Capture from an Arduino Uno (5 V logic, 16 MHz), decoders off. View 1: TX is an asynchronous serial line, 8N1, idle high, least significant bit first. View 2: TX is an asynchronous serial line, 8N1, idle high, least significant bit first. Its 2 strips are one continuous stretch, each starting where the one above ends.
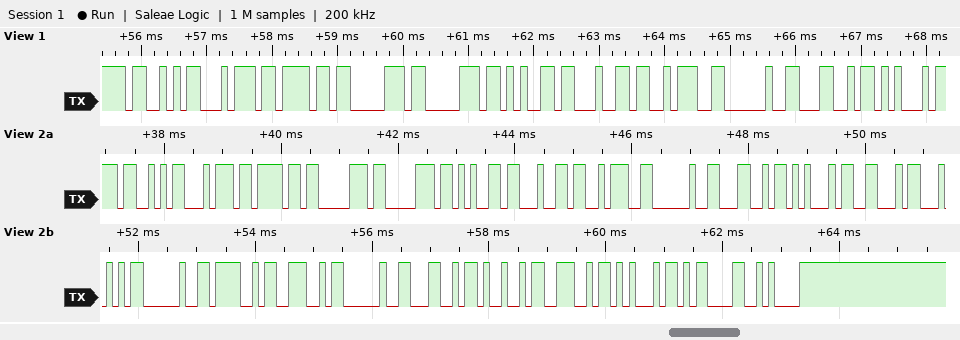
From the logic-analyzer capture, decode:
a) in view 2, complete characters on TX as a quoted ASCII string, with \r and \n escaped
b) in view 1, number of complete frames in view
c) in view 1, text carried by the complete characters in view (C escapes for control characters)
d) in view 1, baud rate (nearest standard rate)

"Stopped: LEFT ON LINE\r\n"
11
"Stopped: LE"
9600 baud
